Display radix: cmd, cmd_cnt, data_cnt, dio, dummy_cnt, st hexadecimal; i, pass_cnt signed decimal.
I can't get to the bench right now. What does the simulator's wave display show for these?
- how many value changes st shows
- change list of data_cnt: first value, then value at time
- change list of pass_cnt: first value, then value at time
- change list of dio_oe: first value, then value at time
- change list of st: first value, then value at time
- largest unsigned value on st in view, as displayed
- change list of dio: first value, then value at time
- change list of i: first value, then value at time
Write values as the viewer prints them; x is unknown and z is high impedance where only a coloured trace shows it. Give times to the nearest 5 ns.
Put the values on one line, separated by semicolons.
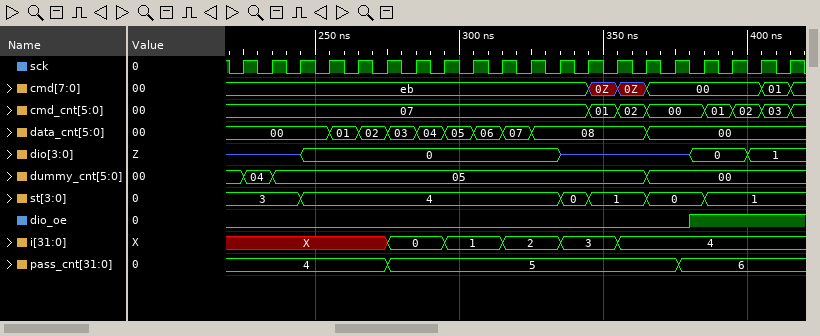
5; 00, 01 at 255 ns, 02 at 265 ns, 03 at 275 ns, 04 at 285 ns, 05 at 295 ns, 06 at 305 ns, 07 at 315 ns, 08 at 325 ns, 00 at 365 ns; 4, 5 at 275 ns, 6 at 375 ns; 0, 1 at 380 ns; 3, 4 at 245 ns, 0 at 335 ns, 1 at 345 ns, 0 at 365 ns, 1 at 385 ns; 4; z, 0 at 245 ns, z at 335 ns, 0 at 380 ns, 1 at 400 ns; X, 0 at 275 ns, 1 at 295 ns, 2 at 315 ns, 3 at 335 ns, 4 at 355 ns
